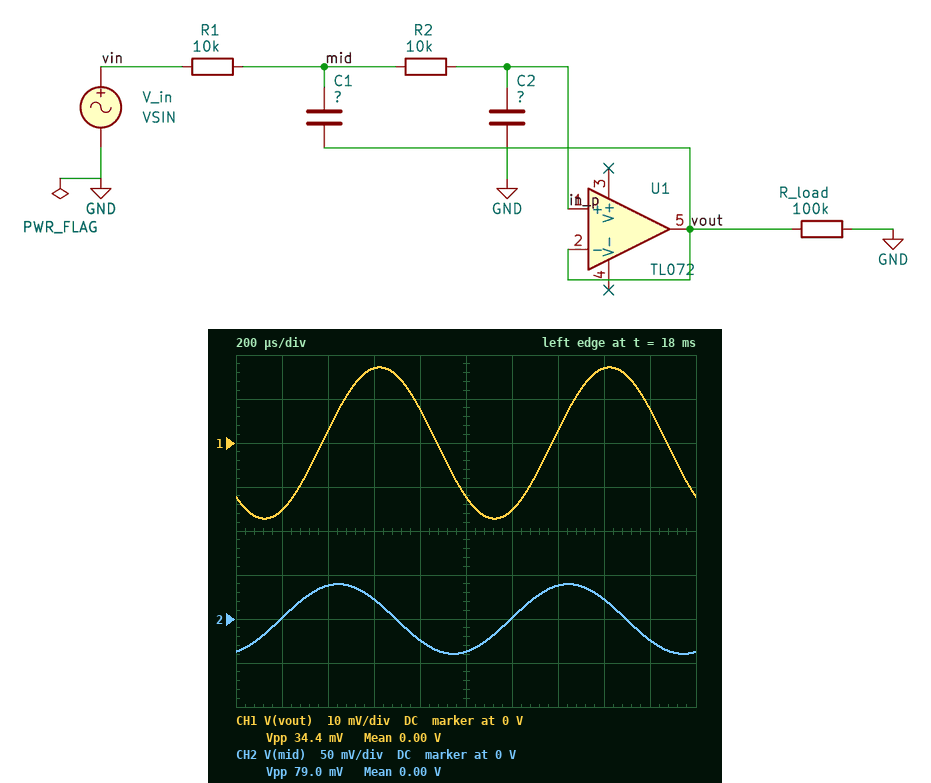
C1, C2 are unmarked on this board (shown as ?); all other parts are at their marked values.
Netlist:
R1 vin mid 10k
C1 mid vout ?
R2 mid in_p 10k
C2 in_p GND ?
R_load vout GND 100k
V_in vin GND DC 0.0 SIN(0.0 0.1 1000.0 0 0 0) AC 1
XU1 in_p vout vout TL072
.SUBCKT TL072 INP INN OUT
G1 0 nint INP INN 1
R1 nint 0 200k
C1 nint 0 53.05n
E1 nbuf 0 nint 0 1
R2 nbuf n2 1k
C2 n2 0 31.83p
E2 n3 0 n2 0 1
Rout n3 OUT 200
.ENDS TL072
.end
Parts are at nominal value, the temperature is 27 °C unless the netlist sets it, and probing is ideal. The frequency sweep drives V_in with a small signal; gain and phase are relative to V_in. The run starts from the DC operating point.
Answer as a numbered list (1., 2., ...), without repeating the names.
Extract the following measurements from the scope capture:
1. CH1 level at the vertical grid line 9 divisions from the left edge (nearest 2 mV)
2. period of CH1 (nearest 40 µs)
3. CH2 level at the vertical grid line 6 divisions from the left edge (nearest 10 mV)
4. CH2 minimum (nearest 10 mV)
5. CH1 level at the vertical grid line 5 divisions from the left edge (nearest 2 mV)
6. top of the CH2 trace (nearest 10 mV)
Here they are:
1. 8 mV
2. 1.00 ms
3. 0 V
4. -40 mV
5. -12 mV
6. 40 mV
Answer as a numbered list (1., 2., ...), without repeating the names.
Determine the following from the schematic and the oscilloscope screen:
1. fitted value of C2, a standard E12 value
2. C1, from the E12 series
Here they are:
1. 33 nF
2. 39 nF
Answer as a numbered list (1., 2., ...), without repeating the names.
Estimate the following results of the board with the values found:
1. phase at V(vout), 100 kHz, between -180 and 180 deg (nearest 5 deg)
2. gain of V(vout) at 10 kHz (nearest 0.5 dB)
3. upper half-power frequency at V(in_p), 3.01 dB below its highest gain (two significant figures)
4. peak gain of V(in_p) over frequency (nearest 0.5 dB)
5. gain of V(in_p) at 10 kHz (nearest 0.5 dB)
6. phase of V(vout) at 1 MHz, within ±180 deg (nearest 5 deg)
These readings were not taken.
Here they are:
1. 90 deg
2. -54.0 dB
3. 320 Hz
4. 0 dB
5. -54.0 dB
6. 80 deg
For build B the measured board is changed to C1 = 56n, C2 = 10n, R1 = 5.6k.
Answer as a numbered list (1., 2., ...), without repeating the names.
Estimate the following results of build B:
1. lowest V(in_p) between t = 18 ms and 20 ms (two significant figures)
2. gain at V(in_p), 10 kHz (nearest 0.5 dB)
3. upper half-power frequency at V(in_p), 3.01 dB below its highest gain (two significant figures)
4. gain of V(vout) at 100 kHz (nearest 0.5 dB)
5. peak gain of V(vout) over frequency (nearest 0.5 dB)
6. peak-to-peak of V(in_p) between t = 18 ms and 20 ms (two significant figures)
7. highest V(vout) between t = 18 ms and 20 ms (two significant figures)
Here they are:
1. -99 mV
2. -42.0 dB
3. 1.1 kHz
4. -58.5 dB
5. 2.0 dB
6. 200 mV
7. 99 mV
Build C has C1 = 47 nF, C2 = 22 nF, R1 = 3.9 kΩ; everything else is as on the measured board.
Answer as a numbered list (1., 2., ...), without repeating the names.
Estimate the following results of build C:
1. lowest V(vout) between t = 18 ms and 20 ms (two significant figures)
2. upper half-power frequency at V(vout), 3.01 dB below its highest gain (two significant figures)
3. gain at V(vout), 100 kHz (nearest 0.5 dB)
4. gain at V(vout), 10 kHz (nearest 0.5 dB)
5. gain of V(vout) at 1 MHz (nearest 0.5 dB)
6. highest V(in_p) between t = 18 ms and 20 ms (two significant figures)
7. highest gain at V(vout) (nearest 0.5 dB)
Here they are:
1. -50 mV
2. 730 Hz
3. -55.5 dB
4. -44.0 dB
5. -35.0 dB
6. 50 mV
7. 0 dB
